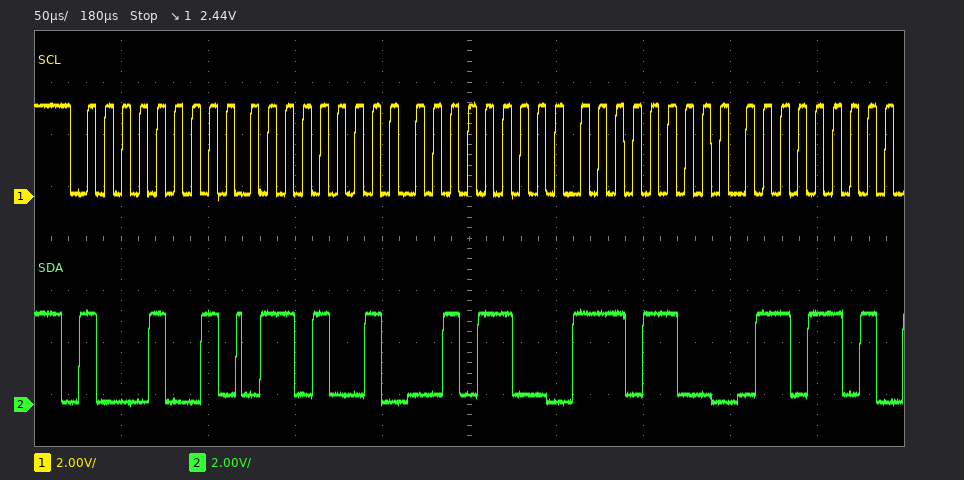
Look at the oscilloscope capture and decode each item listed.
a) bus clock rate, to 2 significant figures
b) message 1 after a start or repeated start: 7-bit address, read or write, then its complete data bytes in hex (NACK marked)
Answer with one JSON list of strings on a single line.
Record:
["100 kHz", "0x44 read: 69 2C EC 6D"]
